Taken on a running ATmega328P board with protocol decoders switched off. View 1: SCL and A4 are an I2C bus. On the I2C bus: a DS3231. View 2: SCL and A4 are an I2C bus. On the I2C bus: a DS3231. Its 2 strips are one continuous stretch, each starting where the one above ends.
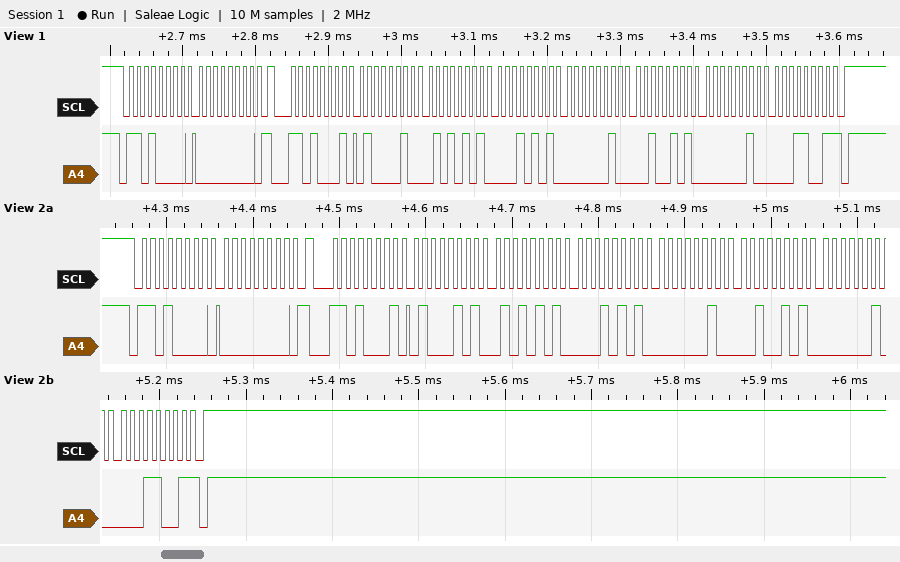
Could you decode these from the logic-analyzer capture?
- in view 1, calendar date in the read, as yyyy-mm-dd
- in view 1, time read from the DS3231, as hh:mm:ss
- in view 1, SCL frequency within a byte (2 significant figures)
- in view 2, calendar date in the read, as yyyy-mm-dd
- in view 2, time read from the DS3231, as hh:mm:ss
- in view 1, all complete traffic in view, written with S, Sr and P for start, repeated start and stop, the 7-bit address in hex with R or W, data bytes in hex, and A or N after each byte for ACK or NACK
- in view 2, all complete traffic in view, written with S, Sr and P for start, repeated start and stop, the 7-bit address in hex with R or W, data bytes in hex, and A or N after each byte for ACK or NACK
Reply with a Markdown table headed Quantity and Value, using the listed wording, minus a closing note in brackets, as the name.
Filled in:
| Quantity | Value |
|---|---|
| in view 1, calendar date in the read, as yyyy-mm-dd | 2019-02-25 |
| in view 1, time read from the DS3231, as hh:mm:ss | 15:55:42 |
| in view 1, SCL frequency within a byte | 100 kHz |
| in view 2, calendar date in the read, as yyyy-mm-dd | 2019-02-25 |
| in view 2, time read from the DS3231, as hh:mm:ss | 15:55:45 |
| in view 1, all complete traffic in view, written with S, Sr and P for start, repeated start and stop, the 7-bit address in hex with R or W, data bytes in hex, and A or N after each byte for ACK or NACK | S 68W A 00 A Sr 68R A 42 A 55 A 15 A 02 A 25 A 02 A 19 N P |
| in view 2, all complete traffic in view, written with S, Sr and P for start, repeated start and stop, the 7-bit address in hex with R or W, data bytes in hex, and A or N after each byte for ACK or NACK | S 68W A 00 A Sr 68R A 45 A 55 A 15 A 02 A 25 A 02 A 19 N P |
